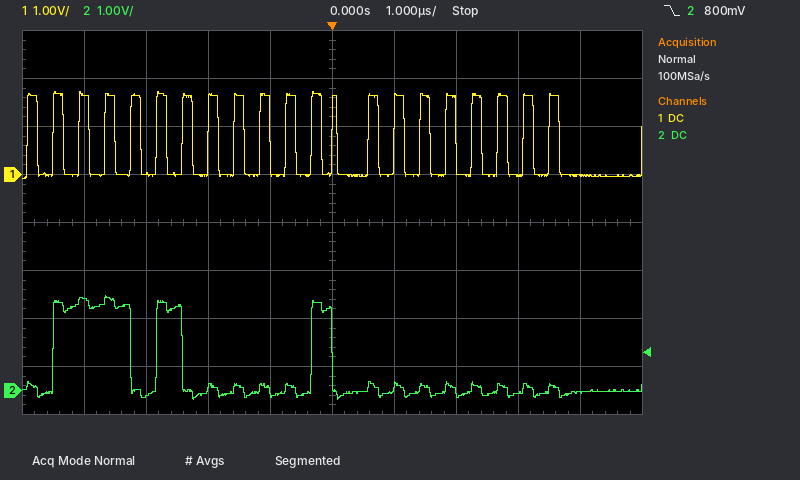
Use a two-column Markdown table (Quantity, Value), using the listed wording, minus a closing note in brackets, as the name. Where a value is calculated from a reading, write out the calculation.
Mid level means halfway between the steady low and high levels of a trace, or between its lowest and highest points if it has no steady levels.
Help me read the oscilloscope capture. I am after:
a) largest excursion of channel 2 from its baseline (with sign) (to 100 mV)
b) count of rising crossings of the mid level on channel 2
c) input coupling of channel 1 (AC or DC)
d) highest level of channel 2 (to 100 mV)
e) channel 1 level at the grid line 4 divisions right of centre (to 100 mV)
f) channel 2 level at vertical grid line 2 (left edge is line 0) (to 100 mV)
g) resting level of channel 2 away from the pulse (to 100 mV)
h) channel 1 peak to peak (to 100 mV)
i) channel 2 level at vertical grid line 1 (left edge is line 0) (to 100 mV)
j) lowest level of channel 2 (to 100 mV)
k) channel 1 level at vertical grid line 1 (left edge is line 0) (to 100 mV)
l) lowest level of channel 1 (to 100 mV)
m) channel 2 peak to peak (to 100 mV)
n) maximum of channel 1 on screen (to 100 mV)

| Quantity | Value |
|---|---|
| largest excursion of channel 2 from its baseline (with sign) | 2.0 V − (0.0 V) = +2.0 V |
| count of rising crossings of the mid level on channel 2 | 3 |
| input coupling of channel 1 | DC |
| highest level of channel 2 | 2.0 V |
| channel 1 level at the grid line 4 divisions right of centre | 0.0 V |
| channel 2 level at vertical grid line 2 (left edge is line 0) | -100 mV |
| resting level of channel 2 away from the pulse | 0.0 V |
| channel 1 peak to peak | 1.7 V − (-100 mV) = 1.8 V |
| channel 2 level at vertical grid line 1 (left edge is line 0) | 1.9 V |
| lowest level of channel 2 | -200 mV |
| channel 1 level at vertical grid line 1 (left edge is line 0) | 1.7 V |
| lowest level of channel 1 | -100 mV |
| channel 2 peak to peak | 2.0 V − (-200 mV) = 2.2 V |
| maximum of channel 1 on screen | 1.7 V |
